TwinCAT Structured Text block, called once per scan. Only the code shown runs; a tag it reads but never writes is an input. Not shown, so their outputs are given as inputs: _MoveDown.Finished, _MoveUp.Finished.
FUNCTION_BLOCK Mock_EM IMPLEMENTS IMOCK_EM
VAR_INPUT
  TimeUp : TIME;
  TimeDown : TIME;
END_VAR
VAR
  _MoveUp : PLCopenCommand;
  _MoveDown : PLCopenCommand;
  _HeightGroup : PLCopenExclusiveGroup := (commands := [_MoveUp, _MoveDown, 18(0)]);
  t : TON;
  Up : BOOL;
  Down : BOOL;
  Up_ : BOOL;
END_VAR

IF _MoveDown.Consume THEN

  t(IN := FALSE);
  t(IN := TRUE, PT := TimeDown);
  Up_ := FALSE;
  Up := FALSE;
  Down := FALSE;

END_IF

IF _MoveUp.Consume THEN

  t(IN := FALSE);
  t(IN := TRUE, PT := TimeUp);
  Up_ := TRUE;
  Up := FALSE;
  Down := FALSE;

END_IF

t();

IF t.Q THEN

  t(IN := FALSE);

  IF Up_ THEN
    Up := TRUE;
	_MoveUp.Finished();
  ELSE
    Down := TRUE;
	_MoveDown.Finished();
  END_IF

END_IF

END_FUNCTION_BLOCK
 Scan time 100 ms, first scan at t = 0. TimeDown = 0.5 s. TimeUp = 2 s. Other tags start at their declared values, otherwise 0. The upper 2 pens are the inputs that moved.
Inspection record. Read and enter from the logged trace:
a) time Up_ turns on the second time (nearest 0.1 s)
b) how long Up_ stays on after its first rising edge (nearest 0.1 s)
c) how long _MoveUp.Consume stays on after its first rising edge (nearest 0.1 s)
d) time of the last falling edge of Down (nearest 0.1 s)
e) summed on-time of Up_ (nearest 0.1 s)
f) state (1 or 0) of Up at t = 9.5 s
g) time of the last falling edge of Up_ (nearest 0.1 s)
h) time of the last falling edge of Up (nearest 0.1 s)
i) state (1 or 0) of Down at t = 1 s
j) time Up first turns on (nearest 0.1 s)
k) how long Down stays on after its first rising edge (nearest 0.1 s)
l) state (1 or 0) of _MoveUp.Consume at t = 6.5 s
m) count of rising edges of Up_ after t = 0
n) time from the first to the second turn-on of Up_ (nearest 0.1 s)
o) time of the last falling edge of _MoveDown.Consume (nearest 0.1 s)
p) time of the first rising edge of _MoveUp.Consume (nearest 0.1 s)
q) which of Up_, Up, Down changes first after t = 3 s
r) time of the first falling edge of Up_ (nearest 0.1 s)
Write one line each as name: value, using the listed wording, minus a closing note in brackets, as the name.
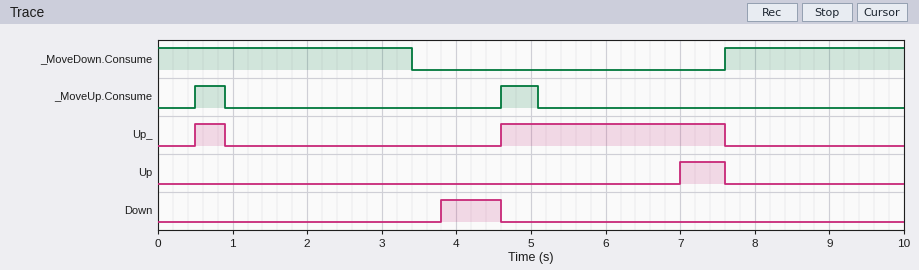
time Up_ turns on the second time: 4.6 s
how long Up_ stays on after its first rising edge: 0.4 s
how long _MoveUp.Consume stays on after its first rising edge: 0.4 s
time of the last falling edge of Down: 4.6 s
summed on-time of Up_: 3.4 s
state (1 or 0) of Up at t = 9.5 s: 0
time of the last falling edge of Up_: 7.6 s
time of the last falling edge of Up: 7.6 s
state (1 or 0) of Down at t = 1 s: 0
time Up first turns on: 7.0 s
how long Down stays on after its first rising edge: 0.8 s
state (1 or 0) of _MoveUp.Consume at t = 6.5 s: 0
count of rising edges of Up_ after t = 0: 2
time from the first to the second turn-on of Up_: 4.1 s
time of the last falling edge of _MoveDown.Consume: 3.4 s
time of the first rising edge of _MoveUp.Consume: 0.5 s
which of Up_, Up, Down changes first after t = 3 s: Down
time of the first falling edge of Up_: 0.9 s
